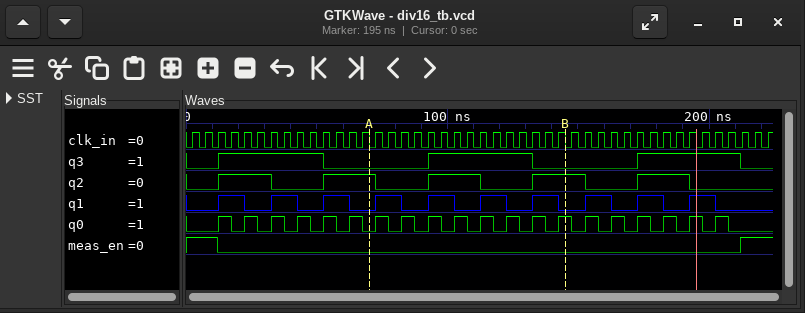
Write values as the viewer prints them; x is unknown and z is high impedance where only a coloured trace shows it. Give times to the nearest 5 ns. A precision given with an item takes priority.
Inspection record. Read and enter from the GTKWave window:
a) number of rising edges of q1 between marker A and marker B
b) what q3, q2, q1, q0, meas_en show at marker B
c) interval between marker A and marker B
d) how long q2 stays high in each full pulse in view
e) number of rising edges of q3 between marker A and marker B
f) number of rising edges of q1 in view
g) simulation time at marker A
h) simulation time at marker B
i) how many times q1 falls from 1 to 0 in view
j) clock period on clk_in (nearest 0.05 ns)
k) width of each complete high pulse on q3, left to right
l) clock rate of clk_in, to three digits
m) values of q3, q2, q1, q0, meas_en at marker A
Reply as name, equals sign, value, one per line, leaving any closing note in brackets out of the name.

number of rising edges of q1 between marker A and marker B = 4
what q3, q2, q1, q0, meas_en show at marker B = q3=0, q2=1, q1=0, q0=1, meas_en=0
interval between marker A and marker B = 75 ns
how long q2 stays high in each full pulse in view = 20 ns, 20 ns, 20 ns, 20 ns, 20 ns
number of rising edges of q3 between marker A and marker B = 1
number of rising edges of q1 in view = 10
simulation time at marker A = 70 ns
simulation time at marker B = 145 ns
how many times q1 falls from 1 to 0 in view = 10
clock period on clk_in = 5 ns
width of each complete high pulse on q3, left to right = 40 ns, 40 ns, 40 ns
clock rate of clk_in, to three digits = 200 MHz
values of q3, q2, q1, q0, meas_en at marker A = q3=0, q2=1, q1=0, q0=0, meas_en=0
